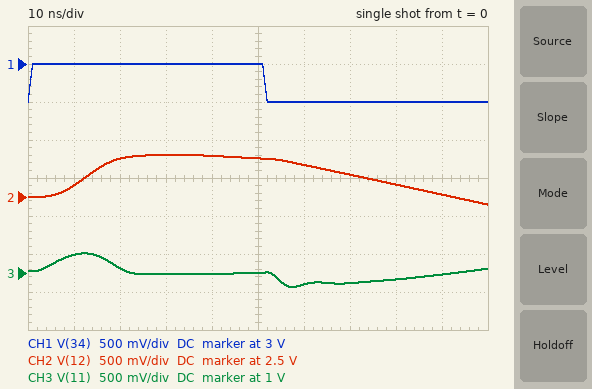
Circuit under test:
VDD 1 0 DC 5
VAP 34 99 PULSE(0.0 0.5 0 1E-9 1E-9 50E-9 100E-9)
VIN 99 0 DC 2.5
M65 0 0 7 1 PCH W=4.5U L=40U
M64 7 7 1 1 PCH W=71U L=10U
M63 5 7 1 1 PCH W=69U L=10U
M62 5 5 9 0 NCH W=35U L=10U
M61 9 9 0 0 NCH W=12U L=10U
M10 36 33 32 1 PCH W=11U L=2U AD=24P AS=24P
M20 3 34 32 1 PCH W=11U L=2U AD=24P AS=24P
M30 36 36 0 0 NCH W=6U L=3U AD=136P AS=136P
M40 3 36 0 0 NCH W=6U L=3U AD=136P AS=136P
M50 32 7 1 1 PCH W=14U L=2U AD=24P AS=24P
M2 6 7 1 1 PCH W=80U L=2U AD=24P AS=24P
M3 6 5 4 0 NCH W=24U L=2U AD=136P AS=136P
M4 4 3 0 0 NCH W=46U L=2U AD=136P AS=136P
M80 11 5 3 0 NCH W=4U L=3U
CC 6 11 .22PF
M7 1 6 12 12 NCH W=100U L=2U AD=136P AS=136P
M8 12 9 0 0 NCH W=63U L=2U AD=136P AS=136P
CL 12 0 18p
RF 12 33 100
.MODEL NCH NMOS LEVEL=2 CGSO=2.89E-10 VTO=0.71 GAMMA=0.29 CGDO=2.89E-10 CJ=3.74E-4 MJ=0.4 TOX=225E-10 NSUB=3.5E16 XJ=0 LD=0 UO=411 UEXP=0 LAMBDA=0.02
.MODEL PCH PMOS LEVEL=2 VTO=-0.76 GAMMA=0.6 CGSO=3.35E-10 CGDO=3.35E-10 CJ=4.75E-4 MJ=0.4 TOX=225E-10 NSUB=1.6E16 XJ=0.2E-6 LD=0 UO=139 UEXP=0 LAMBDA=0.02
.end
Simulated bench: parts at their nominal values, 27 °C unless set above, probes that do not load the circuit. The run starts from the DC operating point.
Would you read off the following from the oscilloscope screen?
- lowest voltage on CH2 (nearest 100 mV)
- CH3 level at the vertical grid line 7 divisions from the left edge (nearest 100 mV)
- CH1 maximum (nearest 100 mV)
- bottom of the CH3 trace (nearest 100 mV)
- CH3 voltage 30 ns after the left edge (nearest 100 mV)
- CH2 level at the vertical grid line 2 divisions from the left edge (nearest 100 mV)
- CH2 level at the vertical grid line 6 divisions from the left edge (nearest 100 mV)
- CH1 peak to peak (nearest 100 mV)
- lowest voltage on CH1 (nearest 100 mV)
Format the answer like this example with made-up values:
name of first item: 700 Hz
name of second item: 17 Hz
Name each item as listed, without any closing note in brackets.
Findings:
lowest voltage on CH2: 2.4 V
CH3 level at the vertical grid line 7 divisions from the left edge: 900 mV
CH1 maximum: 3.0 V
bottom of the CH3 trace: 800 mV
CH3 voltage 30 ns after the left edge: 1.0 V
CH2 level at the vertical grid line 2 divisions from the left edge: 3.0 V
CH2 level at the vertical grid line 6 divisions from the left edge: 2.9 V
CH1 peak to peak: 500 mV
lowest voltage on CH1: 2.5 V
